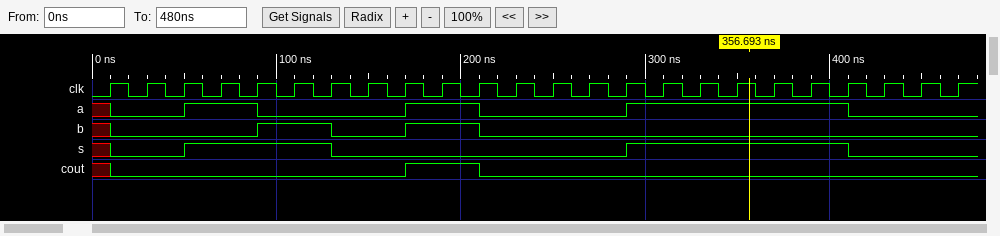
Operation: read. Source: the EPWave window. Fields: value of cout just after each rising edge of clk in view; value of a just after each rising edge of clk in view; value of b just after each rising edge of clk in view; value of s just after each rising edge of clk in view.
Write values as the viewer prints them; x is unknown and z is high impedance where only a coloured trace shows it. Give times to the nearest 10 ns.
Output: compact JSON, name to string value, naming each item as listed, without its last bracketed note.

{"value of cout just after each rising edge of clk in view": "0 0 0 0 0 0 0 0 1 1 0 0 0 0 0 0 0 0 0 0 0 0 0 0", "value of a just after each rising edge of clk in view": "0 0 1 1 0 0 0 0 1 1 0 0 0 0 1 1 1 1 1 1 0 0 0 0", "value of b just after each rising edge of clk in view": "0 0 0 0 1 1 0 0 1 1 0 0 0 0 0 0 0 0 0 0 0 0 0 0", "value of s just after each rising edge of clk in view": "0 0 1 1 1 1 0 0 0 0 0 0 0 0 1 1 1 1 1 1 0 0 0 0"}
